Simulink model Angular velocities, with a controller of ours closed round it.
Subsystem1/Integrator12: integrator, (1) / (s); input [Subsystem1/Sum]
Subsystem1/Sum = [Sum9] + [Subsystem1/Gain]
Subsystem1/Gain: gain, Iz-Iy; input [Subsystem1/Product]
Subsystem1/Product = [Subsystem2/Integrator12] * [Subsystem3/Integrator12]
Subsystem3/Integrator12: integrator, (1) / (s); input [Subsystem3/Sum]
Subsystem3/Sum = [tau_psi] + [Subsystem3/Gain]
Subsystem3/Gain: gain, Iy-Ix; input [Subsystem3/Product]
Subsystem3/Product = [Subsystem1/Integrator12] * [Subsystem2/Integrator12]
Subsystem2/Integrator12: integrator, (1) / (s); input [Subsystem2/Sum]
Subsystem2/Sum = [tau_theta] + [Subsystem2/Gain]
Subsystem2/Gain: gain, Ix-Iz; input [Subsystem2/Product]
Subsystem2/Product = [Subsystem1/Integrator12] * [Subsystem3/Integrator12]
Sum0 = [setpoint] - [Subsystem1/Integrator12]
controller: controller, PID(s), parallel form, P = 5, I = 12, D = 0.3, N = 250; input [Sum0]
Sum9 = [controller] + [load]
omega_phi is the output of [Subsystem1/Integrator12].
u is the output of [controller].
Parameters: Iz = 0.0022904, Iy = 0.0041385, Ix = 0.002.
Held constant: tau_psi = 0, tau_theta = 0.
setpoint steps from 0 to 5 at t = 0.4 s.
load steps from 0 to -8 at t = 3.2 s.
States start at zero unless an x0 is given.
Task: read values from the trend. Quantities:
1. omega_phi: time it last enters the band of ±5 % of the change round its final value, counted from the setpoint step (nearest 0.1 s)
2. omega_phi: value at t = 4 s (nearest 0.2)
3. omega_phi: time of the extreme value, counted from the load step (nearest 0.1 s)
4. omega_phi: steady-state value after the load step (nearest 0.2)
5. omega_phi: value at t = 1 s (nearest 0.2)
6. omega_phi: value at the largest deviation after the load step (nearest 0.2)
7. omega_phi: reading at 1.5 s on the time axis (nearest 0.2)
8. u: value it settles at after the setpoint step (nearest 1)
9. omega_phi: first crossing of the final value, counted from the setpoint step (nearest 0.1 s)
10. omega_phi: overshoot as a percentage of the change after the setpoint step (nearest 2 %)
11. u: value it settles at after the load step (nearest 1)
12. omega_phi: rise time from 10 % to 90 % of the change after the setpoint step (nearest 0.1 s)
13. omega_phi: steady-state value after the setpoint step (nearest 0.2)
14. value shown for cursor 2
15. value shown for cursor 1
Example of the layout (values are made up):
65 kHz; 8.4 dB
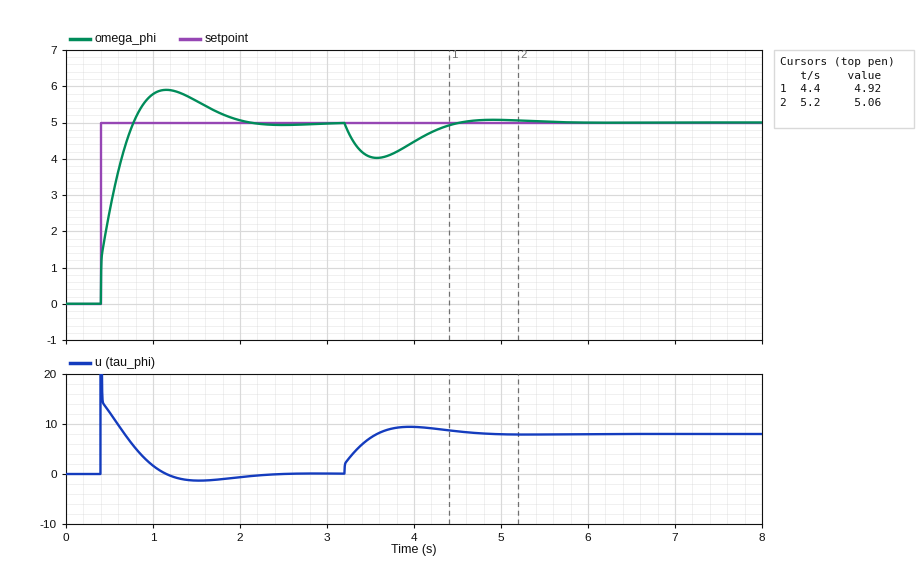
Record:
1.4 s; 4.4; 0.4 s; 5.0; 5.8; 4.0; 5.6; 0; 0.4 s; 18 %; 8; 0.3 s; 5.0; 5.06; 4.92
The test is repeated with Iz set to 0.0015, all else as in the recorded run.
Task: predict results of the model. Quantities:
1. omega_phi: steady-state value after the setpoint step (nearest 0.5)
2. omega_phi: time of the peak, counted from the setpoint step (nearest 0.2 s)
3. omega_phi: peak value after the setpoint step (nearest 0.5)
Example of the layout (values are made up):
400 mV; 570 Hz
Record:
5.0; 0.8 s; 6.0
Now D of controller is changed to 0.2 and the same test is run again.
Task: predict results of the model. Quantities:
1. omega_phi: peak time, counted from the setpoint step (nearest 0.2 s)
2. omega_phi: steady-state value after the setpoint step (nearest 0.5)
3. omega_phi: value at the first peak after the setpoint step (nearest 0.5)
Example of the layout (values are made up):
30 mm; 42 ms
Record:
0.8 s; 5.0; 6.0
